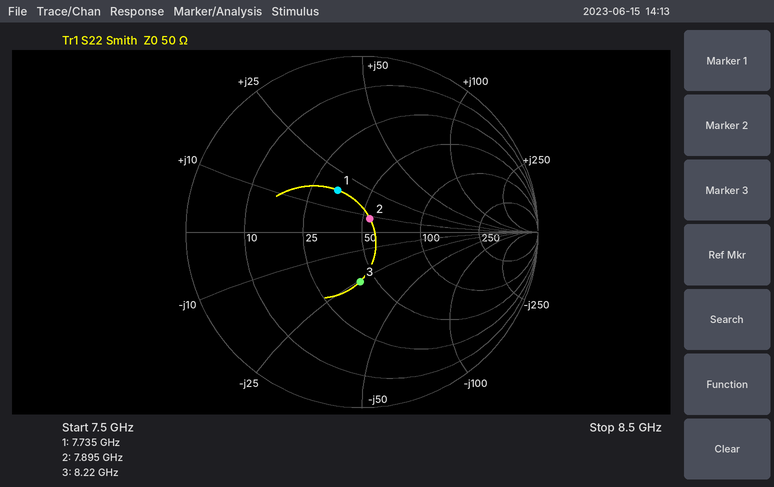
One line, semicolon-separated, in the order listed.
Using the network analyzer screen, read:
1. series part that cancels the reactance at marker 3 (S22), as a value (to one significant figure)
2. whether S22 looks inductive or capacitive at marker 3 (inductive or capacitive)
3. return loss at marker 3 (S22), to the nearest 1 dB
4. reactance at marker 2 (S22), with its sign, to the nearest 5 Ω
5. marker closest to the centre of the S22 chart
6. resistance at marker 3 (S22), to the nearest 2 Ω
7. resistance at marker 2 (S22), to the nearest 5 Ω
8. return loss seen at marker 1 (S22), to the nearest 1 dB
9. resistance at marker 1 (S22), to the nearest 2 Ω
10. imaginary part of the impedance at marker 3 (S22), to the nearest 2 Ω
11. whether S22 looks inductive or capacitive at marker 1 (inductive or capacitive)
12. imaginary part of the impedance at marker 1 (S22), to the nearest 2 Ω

500 pH; capacitive; 11 dB; +10 Ω; marker 2; 42 Ω; 55 Ω; 11 dB; 34 Ω; -26 Ω; inductive; +18 Ω
